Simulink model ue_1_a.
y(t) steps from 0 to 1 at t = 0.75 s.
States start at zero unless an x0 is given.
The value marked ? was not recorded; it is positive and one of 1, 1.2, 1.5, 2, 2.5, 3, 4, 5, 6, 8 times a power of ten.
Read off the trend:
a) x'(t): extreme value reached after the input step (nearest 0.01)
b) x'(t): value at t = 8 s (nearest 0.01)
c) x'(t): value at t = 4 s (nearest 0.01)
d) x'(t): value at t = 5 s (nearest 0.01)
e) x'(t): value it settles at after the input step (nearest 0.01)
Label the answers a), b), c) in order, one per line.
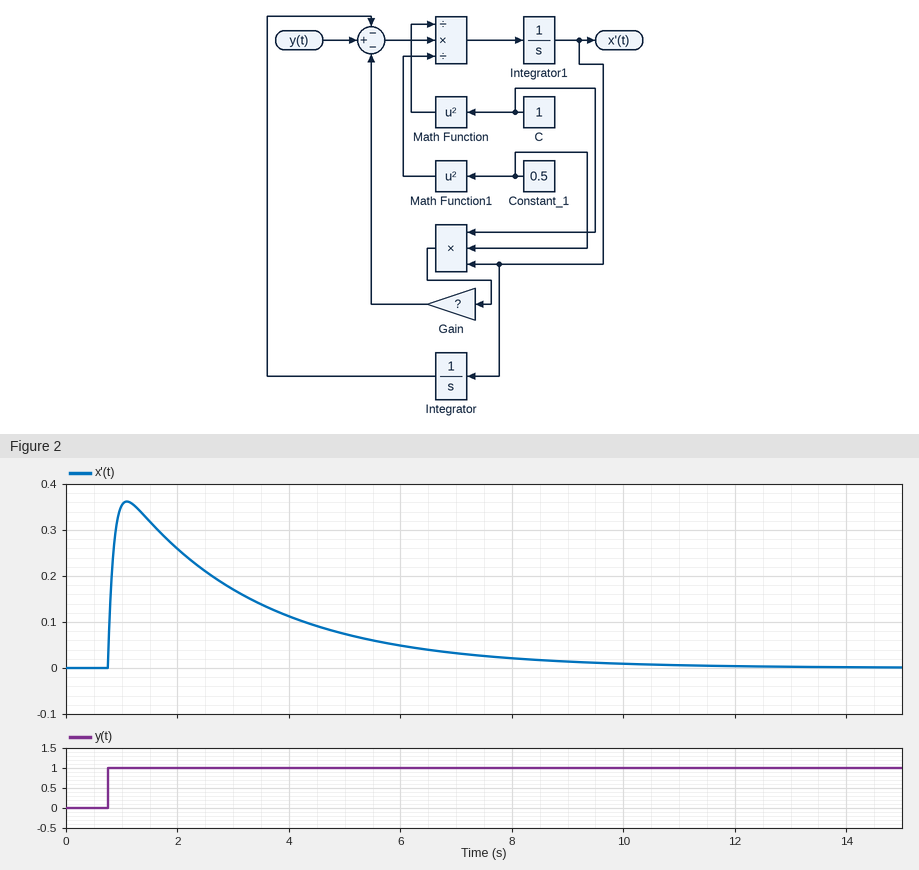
a) 0.36
b) 0.02
c) 0.11
d) 0.07
e) 0.00
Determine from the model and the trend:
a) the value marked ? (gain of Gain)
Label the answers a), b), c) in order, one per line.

a) 5
